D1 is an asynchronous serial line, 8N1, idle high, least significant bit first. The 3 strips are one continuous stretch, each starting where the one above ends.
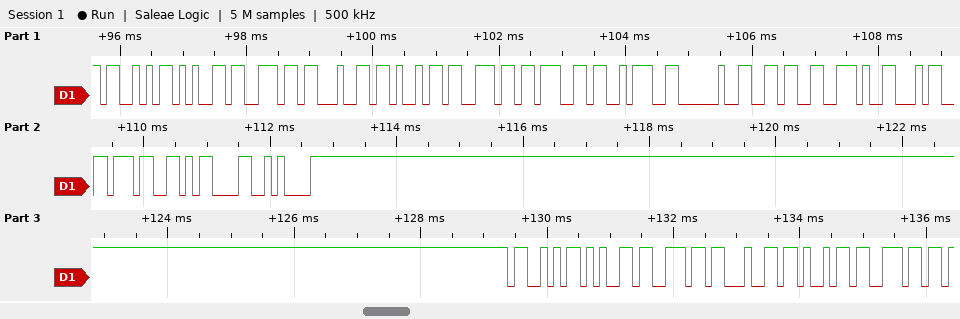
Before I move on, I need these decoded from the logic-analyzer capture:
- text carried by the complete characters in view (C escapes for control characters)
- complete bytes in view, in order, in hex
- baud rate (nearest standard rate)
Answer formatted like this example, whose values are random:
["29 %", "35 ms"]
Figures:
["\"Sending: 6.47\\r\\nSendin\"", "53 65 6E 64 69 6E 67 3A 20 36 2E 34 37 0D 0A 53 65 6E 64 69 6E", "9600 baud"]
